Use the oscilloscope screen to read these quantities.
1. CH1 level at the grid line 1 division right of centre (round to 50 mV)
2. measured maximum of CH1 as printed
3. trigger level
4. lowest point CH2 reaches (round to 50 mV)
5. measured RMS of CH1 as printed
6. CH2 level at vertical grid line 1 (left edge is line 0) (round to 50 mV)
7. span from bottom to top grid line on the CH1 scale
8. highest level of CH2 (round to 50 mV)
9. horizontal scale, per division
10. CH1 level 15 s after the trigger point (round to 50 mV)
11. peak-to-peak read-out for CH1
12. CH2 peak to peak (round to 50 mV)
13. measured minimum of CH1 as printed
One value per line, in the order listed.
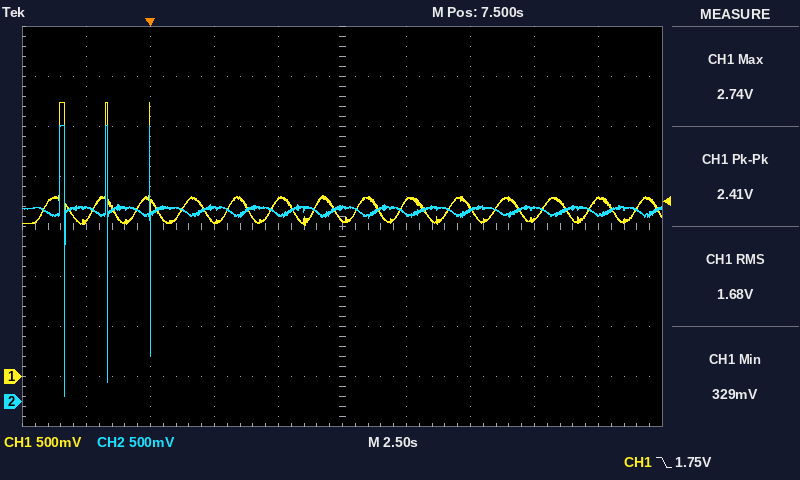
1.75 V
2.74 V
1.75 V
50 mV
1.68 V
1.95 V
4 V
2.75 V
2.5 s
1.55 V
2.41 V
2.70 V
329 mV
